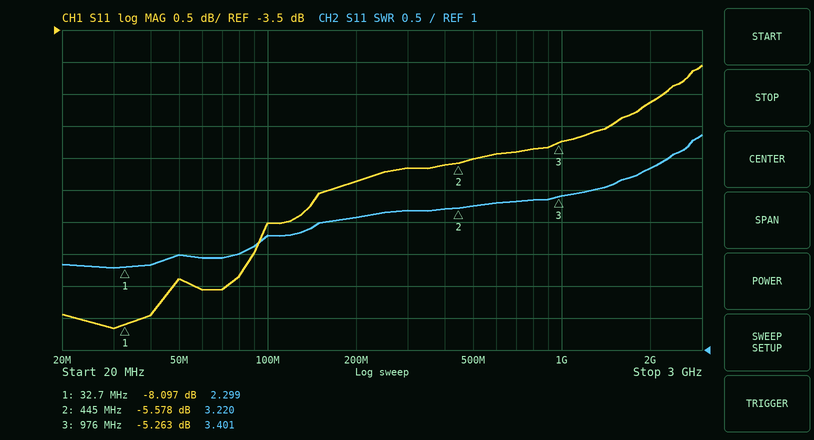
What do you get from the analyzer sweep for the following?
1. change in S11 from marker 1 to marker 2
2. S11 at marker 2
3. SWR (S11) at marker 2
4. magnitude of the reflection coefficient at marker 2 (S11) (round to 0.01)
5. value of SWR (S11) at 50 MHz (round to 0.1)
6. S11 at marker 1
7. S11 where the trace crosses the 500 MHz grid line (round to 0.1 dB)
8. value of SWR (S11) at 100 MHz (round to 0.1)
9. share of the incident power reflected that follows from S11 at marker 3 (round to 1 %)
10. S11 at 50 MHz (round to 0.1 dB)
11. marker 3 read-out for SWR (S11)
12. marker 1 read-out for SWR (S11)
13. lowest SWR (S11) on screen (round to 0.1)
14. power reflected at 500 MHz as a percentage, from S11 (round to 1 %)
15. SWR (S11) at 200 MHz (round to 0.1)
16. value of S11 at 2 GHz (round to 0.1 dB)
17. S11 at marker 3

2.519 dB
-5.578 dB
3.220
0.53
2.5
-8.097 dB
-5.5 dB
2.8
30 %
-7.4 dB
3.401
2.299
2.3
28 %
3.1
-4.6 dB
-5.263 dB
